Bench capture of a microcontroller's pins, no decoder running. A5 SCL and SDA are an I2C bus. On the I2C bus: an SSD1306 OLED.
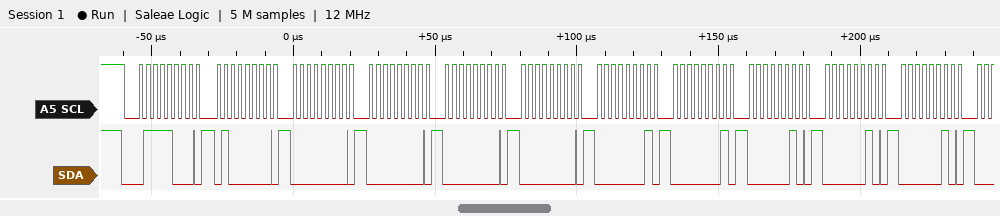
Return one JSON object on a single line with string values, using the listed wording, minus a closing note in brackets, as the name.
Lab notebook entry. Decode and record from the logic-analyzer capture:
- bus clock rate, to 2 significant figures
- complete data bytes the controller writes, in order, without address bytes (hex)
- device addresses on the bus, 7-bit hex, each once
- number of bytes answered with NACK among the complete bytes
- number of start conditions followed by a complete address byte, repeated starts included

{"bus clock rate, to 2 significant figures": "400 kHz", "complete data bytes the controller writes, in order, without address bytes": "40 00 00 00 00 01 01 02 02 02", "device addresses on the bus, 7-bit hex, each once": "0x3C", "number of bytes answered with NACK among the complete bytes": "0", "number of start conditions followed by a complete address byte, repeated starts included": "1"}
